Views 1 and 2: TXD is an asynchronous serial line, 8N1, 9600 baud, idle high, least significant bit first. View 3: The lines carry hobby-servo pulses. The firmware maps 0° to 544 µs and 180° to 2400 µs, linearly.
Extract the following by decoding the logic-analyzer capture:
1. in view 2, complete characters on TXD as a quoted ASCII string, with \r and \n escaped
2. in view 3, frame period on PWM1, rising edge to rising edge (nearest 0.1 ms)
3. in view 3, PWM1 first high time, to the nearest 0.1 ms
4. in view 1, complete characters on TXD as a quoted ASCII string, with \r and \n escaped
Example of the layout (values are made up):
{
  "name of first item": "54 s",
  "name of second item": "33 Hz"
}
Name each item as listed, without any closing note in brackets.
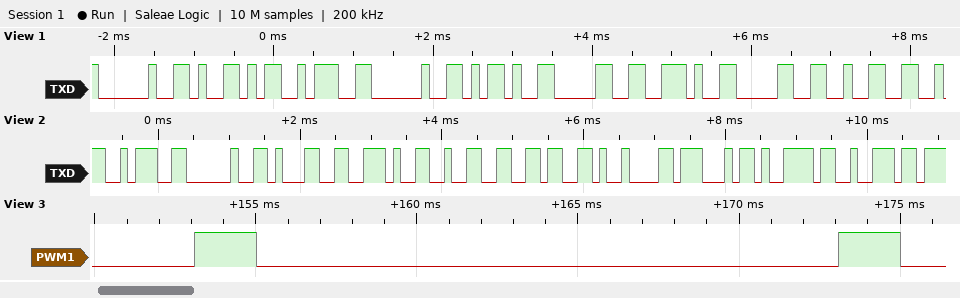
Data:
{
  "in view 2, complete characters on TXD as a quoted ASCII string, with \\r and \\n escaped": "\": 1.26\\tGyr\"",
  "in view 3, frame period on PWM1, rising edge to rising edge": "20.0 ms",
  "in view 3, PWM1 first high time, to the nearest 0.1 ms": "1.9 ms",
  "in view 1, complete characters on TXD as a quoted ASCII string, with \\r and \\n escaped": "\" Y: -0.02\""
}
